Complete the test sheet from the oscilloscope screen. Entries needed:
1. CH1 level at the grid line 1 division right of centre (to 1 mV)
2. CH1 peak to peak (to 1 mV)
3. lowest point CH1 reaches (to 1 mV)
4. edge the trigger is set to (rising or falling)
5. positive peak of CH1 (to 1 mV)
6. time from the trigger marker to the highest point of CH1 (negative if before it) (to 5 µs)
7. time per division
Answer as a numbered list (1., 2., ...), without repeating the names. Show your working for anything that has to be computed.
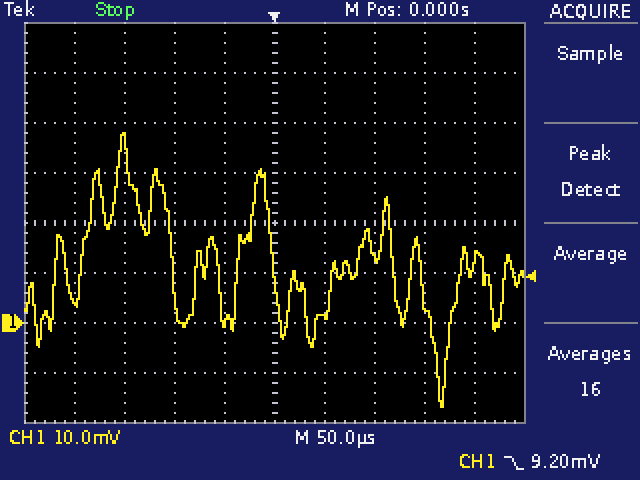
1. 2 mV
2. 38 mV − (-17 mV) = 55 mV
3. -17 mV
4. falling
5. 38 mV
6. -150 µs
7. 50 µs
